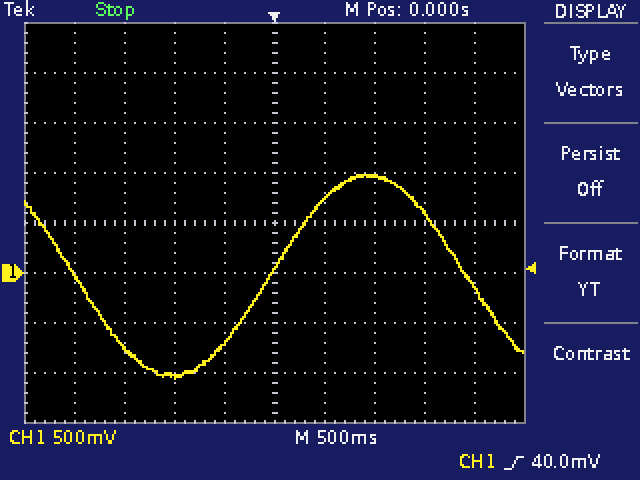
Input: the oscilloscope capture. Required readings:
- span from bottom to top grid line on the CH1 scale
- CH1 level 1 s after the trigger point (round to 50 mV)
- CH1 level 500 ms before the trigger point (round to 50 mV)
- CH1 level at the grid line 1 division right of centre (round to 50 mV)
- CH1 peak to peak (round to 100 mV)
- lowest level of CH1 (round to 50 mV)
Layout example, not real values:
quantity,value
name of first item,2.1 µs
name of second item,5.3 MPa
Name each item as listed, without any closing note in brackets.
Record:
quantity,value
span from bottom to top grid line on the CH1 scale,4 V
CH1 level 1 s after the trigger point,950 mV
CH1 level 500 ms before the trigger point,-700 mV
CH1 level at the grid line 1 division right of centre,750 mV
CH1 peak to peak,2.00 V
lowest level of CH1,-1.05 V
